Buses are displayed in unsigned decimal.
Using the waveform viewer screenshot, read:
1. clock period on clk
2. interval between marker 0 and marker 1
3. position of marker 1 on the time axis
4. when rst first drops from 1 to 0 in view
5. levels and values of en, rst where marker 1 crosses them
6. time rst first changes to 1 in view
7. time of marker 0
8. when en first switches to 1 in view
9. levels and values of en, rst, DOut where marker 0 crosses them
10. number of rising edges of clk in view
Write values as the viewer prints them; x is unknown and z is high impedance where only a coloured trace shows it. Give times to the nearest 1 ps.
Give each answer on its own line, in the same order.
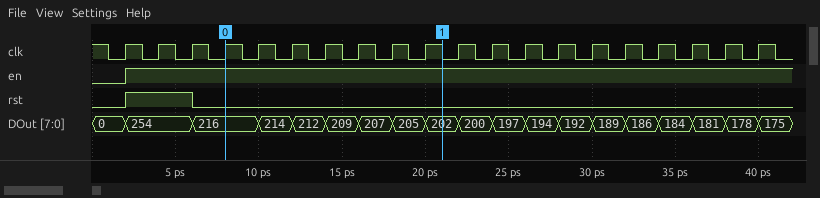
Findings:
2 ps
13 ps
21 ps
6 ps
en=1, rst=0
2 ps
8 ps
2 ps
en=1, rst=0, DOut=216
20
